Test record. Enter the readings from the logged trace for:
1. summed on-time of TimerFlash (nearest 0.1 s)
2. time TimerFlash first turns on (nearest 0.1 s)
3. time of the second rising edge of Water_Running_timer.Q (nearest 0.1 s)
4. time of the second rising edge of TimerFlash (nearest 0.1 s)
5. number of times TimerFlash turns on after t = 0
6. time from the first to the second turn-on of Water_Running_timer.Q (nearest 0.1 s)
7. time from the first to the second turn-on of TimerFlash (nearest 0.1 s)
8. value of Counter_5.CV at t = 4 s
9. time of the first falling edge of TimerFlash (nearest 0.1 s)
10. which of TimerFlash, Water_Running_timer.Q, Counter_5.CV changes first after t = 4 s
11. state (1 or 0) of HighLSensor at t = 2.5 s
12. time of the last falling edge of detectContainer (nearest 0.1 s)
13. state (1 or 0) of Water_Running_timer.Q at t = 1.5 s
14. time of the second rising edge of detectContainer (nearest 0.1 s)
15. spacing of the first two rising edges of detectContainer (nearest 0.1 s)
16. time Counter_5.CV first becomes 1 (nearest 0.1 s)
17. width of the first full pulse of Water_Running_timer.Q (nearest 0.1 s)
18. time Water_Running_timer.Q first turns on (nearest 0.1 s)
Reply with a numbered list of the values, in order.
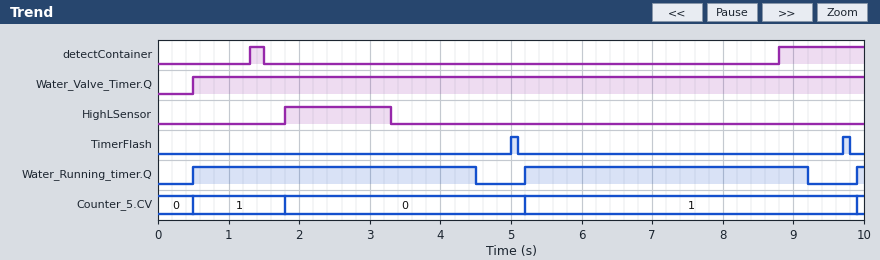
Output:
1. 0.2 s
2. 5.0 s
3. 5.2 s
4. 9.7 s
5. 2
6. 4.7 s
7. 4.7 s
8. 0
9. 5.1 s
10. Water_Running_timer.Q
11. 1
12. 1.5 s
13. 1
14. 8.8 s
15. 7.5 s
16. 0.5 s
17. 4.0 s
18. 0.5 s
